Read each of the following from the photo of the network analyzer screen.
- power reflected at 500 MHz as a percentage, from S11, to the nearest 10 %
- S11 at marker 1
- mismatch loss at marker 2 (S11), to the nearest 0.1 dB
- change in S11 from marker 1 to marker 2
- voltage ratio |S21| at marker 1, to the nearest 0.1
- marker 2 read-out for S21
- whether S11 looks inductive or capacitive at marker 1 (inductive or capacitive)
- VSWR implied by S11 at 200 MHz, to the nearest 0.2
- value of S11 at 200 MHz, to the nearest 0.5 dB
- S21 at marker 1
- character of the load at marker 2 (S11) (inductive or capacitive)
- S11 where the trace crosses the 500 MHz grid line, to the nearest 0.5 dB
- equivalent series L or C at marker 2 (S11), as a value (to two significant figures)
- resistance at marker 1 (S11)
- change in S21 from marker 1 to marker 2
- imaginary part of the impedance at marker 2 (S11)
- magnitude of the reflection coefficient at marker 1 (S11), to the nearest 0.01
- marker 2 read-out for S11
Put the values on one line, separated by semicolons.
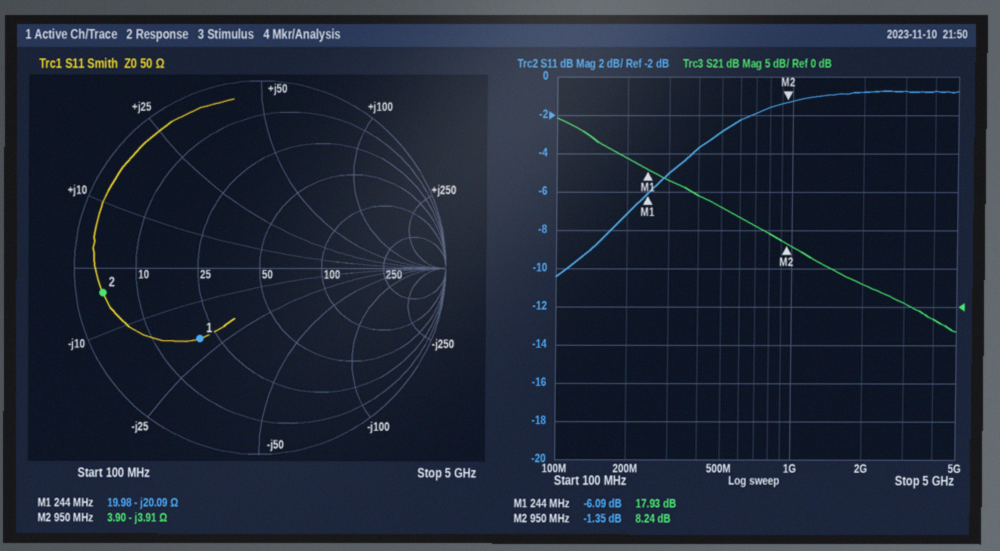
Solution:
50 %; -6.09 dB; 5.7 dB; 4.74 dB; 7.9; 8.24 dB; capacitive; 2.6; -7.0 dB; 17.93 dB; capacitive; -3.0 dB; 43 pF; 19.98 Ω; -9.69 dB; -3.91 Ω; 0.50; -1.35 dB
